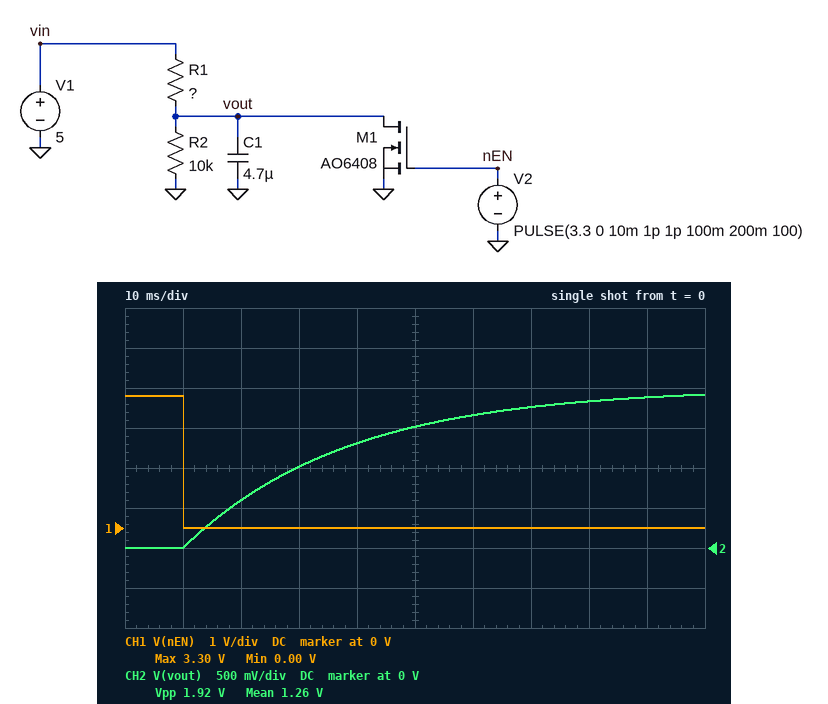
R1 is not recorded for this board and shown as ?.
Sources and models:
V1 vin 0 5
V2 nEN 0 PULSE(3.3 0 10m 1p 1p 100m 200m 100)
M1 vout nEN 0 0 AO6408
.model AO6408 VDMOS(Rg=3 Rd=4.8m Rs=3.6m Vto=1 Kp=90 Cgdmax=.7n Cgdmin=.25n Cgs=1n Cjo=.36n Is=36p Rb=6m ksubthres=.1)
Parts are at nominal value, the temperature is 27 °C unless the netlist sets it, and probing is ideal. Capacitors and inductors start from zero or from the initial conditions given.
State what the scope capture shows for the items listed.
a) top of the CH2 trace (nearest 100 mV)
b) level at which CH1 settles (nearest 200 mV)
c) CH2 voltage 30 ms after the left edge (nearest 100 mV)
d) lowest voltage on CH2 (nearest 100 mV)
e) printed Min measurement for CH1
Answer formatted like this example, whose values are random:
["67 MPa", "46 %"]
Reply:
["1.9 V", "0 V", "1.0 V", "0 V", "0.00 V"]
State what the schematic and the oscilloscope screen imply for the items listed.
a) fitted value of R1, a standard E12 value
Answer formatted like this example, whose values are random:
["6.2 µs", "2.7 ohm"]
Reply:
["15 kΩ"]
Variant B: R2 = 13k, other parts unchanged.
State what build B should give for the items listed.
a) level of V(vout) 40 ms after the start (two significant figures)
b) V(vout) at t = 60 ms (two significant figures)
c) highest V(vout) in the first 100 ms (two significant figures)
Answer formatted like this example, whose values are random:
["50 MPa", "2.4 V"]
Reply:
["1.4 V", "1.8 V", "2.2 V"]
